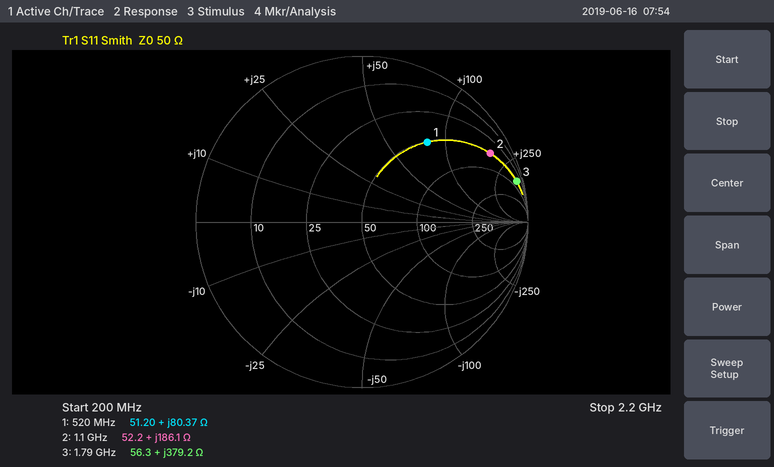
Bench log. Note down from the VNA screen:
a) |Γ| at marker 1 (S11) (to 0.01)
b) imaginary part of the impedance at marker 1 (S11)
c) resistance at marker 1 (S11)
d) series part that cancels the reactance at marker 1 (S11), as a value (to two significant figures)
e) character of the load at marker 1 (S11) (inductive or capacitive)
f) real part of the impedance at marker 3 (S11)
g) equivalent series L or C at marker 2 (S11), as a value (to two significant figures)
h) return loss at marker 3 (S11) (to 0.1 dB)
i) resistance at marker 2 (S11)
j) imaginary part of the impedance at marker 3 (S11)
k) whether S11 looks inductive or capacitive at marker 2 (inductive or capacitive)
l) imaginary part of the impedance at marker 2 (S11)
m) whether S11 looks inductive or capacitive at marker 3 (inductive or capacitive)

0.62
+80.37 Ω
51.20 Ω
3.8 pF
inductive
56.3 Ω
27 nH
0.3 dB
52.2 Ω
+379.2 Ω
inductive
+186.1 Ω
inductive
